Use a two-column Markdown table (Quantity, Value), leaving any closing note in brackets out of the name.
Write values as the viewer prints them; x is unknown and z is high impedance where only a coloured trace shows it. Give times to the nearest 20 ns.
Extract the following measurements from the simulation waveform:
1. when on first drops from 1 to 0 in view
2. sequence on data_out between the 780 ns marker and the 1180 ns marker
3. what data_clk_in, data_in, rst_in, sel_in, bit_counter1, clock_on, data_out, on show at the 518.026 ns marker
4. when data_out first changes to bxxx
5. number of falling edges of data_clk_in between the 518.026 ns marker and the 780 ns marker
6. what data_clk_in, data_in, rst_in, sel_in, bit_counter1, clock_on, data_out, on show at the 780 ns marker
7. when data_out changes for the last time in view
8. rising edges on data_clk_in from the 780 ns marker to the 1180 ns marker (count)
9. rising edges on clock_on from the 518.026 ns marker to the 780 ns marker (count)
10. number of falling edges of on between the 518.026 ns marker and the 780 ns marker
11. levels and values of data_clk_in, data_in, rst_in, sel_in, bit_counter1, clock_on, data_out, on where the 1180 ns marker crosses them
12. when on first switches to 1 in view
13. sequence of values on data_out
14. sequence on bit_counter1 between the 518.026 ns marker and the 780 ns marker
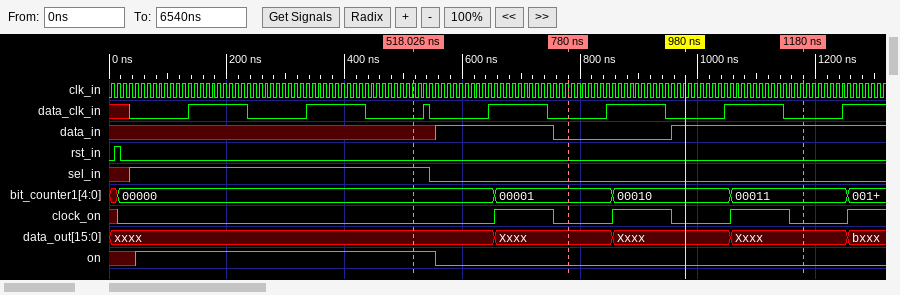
| Quantity | Value |
|---|---|
| when on first drops from 1 to 0 in view | 560 ns |
| sequence on data_out between the 780 ns marker and the 1180 ns marker | Xxxx, Xxxx, Xxxx |
| what data_clk_in, data_in, rst_in, sel_in, bit_counter1, clock_on, data_out, on show at the 518.026 ns marker | data_clk_in=0, data_in=x, rst_in=0, sel_in=1, bit_counter1=00000, clock_on=0, data_out=xxxx, on=1 |
| when data_out first changes to bxxx | 1260 ns |
| number of falling edges of data_clk_in between the 518.026 ns marker and the 780 ns marker | 2 |
| what data_clk_in, data_in, rst_in, sel_in, bit_counter1, clock_on, data_out, on show at the 780 ns marker | data_clk_in=0, data_in=0, rst_in=0, sel_in=0, bit_counter1=00001, clock_on=0, data_out=Xxxx, on=0 |
| when data_out changes for the last time in view | 1260 ns |
| rising edges on data_clk_in from the 780 ns marker to the 1180 ns marker | 2 |
| rising edges on clock_on from the 518.026 ns marker to the 780 ns marker | 1 |
| number of falling edges of on between the 518.026 ns marker and the 780 ns marker | 1 |
| levels and values of data_clk_in, data_in, rst_in, sel_in, bit_counter1, clock_on, data_out, on where the 1180 ns marker crosses them | data_clk_in=0, data_in=1, rst_in=0, sel_in=0, bit_counter1=00011, clock_on=0, data_out=Xxxx, on=0 |
| when on first switches to 1 in view | 40 ns |
| sequence of values on data_out | xxxx, Xxxx, Xxxx, Xxxx, bxxx |
| sequence on bit_counter1 between the 518.026 ns marker and the 780 ns marker | 00000, 00001 |
